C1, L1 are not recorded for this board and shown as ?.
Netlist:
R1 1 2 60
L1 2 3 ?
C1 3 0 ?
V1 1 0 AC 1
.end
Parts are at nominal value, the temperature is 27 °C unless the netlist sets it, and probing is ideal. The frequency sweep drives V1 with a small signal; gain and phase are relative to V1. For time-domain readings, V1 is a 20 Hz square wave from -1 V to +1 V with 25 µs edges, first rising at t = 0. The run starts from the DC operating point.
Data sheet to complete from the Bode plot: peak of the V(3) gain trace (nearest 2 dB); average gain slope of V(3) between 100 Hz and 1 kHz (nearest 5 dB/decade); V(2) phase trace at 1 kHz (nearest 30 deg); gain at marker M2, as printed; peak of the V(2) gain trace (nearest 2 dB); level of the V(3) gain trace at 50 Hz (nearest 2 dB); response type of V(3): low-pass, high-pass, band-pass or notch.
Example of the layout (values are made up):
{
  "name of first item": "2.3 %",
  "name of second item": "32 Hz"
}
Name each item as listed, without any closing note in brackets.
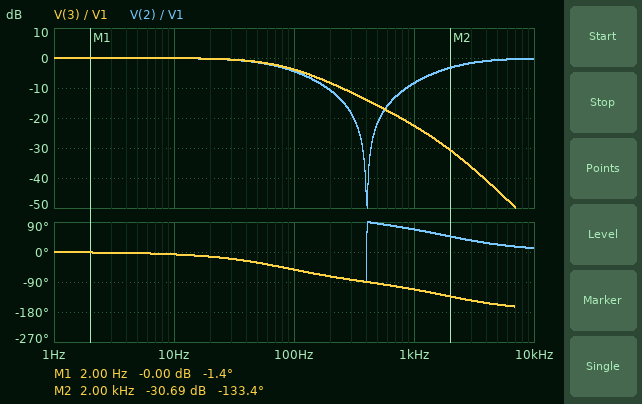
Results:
{
  "peak of the V(3) gain trace": "0 dB",
  "average gain slope of V(3) between 100 Hz and 1 kHz": "-20 dB/decade",
  "V(2) phase trace at 1 kHz": "60 deg",
  "gain at marker M2, as printed": "-30.69 dB",
  "peak of the V(2) gain trace": "0 dB",
  "level of the V(3) gain trace at 50 Hz": "-2 dB",
  "response type of V(3): low-pass, high-pass, band-pass or notch": "low-pass"
}
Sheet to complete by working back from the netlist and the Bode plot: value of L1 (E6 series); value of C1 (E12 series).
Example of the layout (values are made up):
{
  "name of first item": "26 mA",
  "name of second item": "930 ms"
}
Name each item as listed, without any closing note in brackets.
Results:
{
  "value of L1": "4.7 mH",
  "value of C1": "33 µF"
}
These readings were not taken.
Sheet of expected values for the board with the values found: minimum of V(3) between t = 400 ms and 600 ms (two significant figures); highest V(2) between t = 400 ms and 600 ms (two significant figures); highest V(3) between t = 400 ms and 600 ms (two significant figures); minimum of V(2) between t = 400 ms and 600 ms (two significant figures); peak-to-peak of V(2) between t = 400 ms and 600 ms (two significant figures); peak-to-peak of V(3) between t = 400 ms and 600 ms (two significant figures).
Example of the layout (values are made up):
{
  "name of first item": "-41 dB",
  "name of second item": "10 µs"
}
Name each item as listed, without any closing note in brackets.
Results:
{
  "minimum of V(3) between t = 400 ms and 600 ms": "-1.0 V",
  "highest V(2) between t = 400 ms and 600 ms": "1.0 V",
  "highest V(3) between t = 400 ms and 600 ms": "1.0 V",
  "minimum of V(2) between t = 400 ms and 600 ms": "-1.0 V",
  "peak-to-peak of V(2) between t = 400 ms and 600 ms": "2.0 V",
  "peak-to-peak of V(3) between t = 400 ms and 600 ms": "2.0 V"
}
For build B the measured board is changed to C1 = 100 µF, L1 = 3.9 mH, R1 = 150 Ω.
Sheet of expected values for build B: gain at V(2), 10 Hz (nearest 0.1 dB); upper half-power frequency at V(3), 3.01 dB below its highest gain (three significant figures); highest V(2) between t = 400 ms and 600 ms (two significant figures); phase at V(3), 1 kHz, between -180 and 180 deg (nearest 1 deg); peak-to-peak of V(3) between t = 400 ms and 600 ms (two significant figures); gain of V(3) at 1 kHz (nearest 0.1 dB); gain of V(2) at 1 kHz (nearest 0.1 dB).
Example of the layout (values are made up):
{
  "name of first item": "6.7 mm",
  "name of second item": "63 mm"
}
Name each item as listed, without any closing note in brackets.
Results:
{
  "gain at V(2), 10 Hz": "-2.8 dB",
  "upper half-power frequency at V(3), 3.01 dB below its highest gain": "10.6 Hz",
  "highest V(2) between t = 400 ms and 600 ms": "680 mV",
  "phase at V(3), 1 kHz, between -180 and 180 deg": "-99 deg",
  "peak-to-peak of V(3) between t = 400 ms and 600 ms": "1.4 V",
  "gain of V(3) at 1 kHz": "-39.6 dB",
  "gain of V(2) at 1 kHz": "-16.4 dB"
}
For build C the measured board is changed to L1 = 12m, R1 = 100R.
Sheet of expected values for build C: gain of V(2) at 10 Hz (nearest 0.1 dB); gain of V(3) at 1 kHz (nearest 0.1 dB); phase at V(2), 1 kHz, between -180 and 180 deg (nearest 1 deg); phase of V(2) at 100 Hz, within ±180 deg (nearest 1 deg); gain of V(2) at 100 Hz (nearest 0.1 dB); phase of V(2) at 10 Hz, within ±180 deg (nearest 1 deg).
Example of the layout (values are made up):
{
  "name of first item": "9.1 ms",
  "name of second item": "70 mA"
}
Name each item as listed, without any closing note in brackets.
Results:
{
  "gain of V(2) at 10 Hz": "-0.2 dB",
  "gain of V(3) at 1 kHz": "-28.1 dB",
  "phase at V(2), 1 kHz, between -180 and 180 deg": "55 deg",
  "phase of V(2) at 100 Hz, within ±180 deg": "-68 deg",
  "gain of V(2) at 100 Hz": "-8.5 dB",
  "phase of V(2) at 10 Hz, within ±180 deg": "-12 deg"
}
